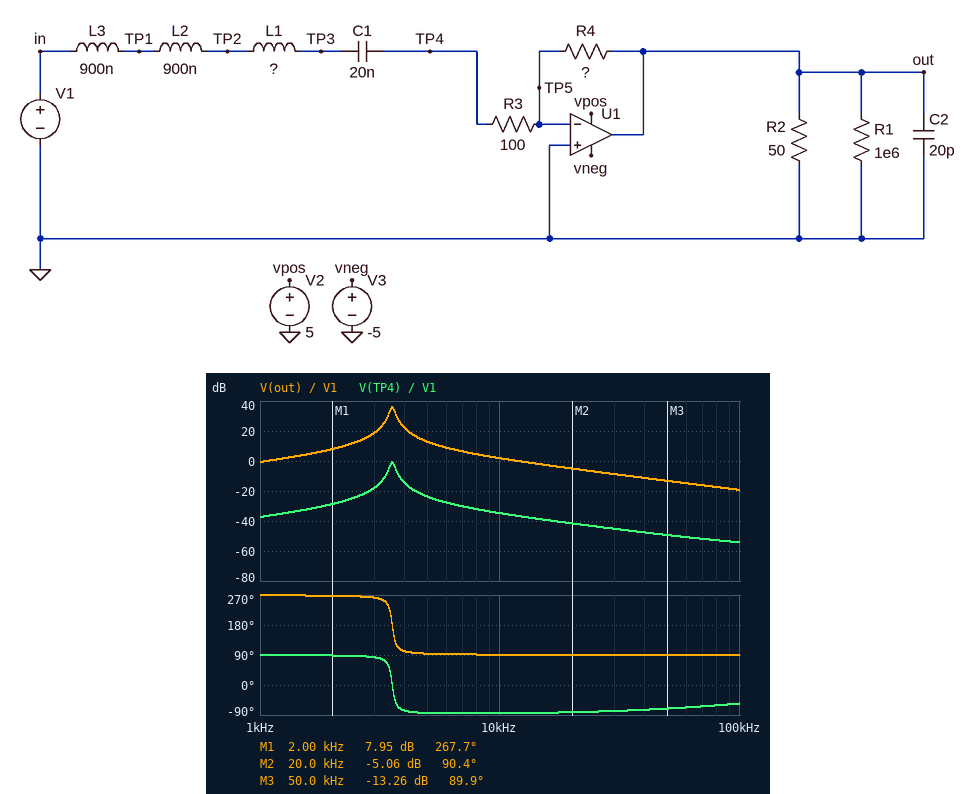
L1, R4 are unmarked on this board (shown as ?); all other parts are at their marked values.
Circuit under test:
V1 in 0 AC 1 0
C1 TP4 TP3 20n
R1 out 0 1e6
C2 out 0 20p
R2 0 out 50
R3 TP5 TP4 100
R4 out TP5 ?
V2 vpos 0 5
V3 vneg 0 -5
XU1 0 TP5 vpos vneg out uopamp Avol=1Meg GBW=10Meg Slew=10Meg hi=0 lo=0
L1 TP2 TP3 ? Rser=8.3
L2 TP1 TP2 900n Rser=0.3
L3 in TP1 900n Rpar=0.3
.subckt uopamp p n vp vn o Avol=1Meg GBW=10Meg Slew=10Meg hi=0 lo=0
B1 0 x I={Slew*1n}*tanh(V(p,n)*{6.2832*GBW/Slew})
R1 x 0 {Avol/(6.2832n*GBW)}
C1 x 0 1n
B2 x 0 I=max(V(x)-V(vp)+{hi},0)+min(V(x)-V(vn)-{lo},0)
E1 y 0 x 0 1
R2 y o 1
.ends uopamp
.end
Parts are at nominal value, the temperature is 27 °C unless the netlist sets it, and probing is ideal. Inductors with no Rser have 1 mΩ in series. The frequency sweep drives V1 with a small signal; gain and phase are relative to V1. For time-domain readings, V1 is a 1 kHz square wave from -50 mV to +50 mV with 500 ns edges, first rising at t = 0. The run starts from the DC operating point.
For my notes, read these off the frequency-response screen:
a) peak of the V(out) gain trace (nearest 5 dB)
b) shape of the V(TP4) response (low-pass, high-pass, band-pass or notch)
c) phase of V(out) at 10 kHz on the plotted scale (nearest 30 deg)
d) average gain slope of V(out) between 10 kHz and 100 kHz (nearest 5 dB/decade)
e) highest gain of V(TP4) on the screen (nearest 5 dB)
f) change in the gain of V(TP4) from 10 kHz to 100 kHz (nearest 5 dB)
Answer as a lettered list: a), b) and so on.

a) 35 dB
b) band-pass
c) 90 deg
d) -20 dB/decade
e) 0 dB
f) -20 dB
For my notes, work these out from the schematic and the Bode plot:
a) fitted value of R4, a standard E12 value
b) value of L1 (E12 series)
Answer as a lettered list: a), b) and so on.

a) 6.8 kΩ
b) 100 mH
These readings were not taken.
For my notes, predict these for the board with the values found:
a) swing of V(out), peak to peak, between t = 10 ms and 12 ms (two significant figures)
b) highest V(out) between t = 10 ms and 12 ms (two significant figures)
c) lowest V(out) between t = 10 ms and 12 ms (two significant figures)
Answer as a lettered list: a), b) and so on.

a) 440 mV
b) 220 mV
c) -220 mV
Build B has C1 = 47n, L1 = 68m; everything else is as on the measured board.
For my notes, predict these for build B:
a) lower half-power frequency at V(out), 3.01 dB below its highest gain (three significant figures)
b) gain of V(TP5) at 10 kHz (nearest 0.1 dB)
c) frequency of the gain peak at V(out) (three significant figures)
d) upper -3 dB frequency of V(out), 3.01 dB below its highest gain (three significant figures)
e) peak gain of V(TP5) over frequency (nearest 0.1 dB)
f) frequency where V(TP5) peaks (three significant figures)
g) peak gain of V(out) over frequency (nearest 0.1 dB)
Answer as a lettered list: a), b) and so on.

a) 2.69 kHz
b) -55.1 dB
c) 2.81 kHz
d) 2.94 kHz
e) -34.9 dB
f) 2.82 kHz
g) 35.9 dB
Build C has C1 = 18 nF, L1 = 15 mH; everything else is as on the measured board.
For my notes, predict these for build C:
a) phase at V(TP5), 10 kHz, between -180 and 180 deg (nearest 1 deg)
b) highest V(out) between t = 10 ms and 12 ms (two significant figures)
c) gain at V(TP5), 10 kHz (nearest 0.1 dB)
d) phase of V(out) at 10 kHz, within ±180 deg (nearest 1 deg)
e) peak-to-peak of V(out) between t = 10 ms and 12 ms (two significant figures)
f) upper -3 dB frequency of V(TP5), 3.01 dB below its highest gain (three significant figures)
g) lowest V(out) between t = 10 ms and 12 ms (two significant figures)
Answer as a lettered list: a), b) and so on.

a) 59 deg
b) 640 mV
c) -25.2 dB
d) 149 deg
e) 1.3 V
f) 10.3 kHz
g) -640 mV
